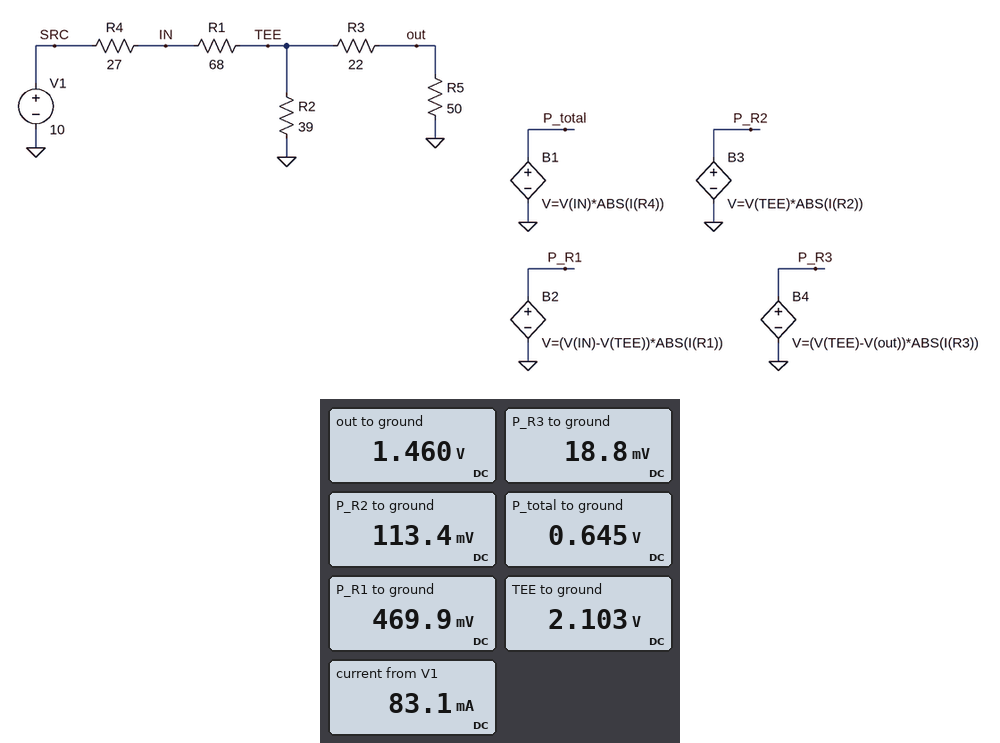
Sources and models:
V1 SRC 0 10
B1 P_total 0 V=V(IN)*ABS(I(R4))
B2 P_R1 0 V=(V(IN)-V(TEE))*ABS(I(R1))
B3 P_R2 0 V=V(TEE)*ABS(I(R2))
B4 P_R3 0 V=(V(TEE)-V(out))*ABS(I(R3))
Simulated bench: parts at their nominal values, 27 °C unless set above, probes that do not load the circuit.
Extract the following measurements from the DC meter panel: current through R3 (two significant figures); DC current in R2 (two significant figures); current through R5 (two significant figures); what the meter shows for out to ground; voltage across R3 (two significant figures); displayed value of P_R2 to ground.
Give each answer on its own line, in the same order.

29 mA
54 mA
29 mA
1.460 V
640 mV
113.4 mV
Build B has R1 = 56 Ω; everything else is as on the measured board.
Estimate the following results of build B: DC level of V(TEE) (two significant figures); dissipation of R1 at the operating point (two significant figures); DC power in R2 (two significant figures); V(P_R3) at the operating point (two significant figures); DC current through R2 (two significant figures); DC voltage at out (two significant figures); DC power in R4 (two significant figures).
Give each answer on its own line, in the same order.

2.3 V
480 mW
140 mW
23 mV
60 mA
1.6 V
230 mW
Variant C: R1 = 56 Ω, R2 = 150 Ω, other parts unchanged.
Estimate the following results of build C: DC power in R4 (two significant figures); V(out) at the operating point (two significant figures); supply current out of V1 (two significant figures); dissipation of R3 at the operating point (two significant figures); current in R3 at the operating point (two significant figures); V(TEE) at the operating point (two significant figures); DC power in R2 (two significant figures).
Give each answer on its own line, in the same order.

160 mW
2.6 V
76 mA
58 mW
51 mA
3.7 V
91 mW
